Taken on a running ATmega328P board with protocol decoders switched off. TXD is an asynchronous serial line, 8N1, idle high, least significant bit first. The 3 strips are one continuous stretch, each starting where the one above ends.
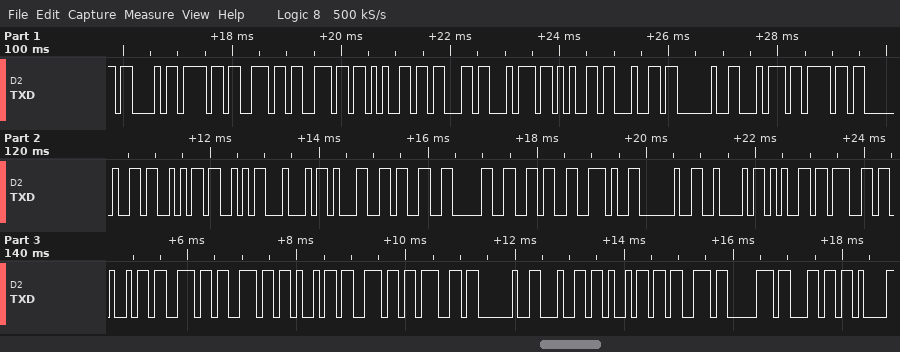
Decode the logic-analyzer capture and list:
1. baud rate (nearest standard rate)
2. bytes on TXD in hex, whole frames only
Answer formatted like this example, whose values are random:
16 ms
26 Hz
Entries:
9600 baud
43 6F 6E 6E 65 63 74 65 64 20 74 6F 20 53 53 44 31 33 30 36 2E 20 42 65 67 69 6E 6E 69 6E 67 20 64 69 73 70 6C
